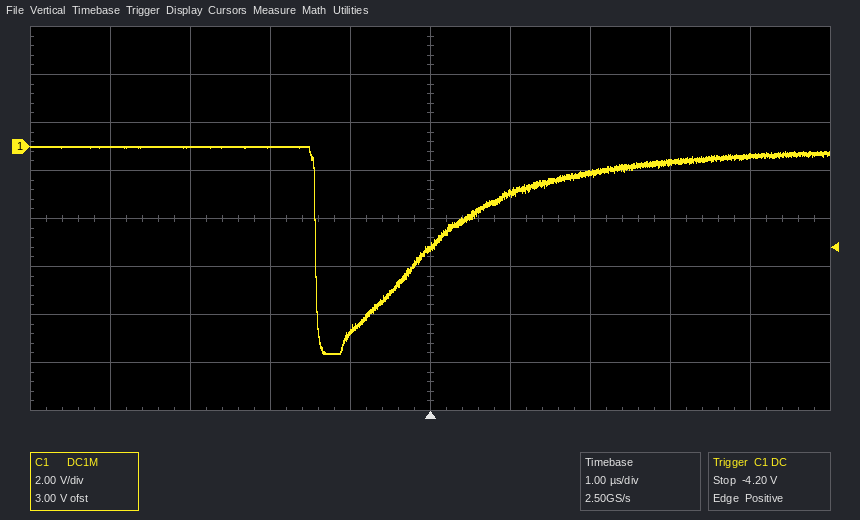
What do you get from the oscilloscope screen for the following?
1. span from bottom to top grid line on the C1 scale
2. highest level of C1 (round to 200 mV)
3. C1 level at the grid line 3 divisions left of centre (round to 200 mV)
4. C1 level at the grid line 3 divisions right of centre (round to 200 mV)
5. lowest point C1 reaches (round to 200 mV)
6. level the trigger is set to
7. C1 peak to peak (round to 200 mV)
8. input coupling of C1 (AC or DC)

16 V
0.0 V
0.0 V
-600 mV
-8.6 V
-4.20 V
8.6 V
DC
